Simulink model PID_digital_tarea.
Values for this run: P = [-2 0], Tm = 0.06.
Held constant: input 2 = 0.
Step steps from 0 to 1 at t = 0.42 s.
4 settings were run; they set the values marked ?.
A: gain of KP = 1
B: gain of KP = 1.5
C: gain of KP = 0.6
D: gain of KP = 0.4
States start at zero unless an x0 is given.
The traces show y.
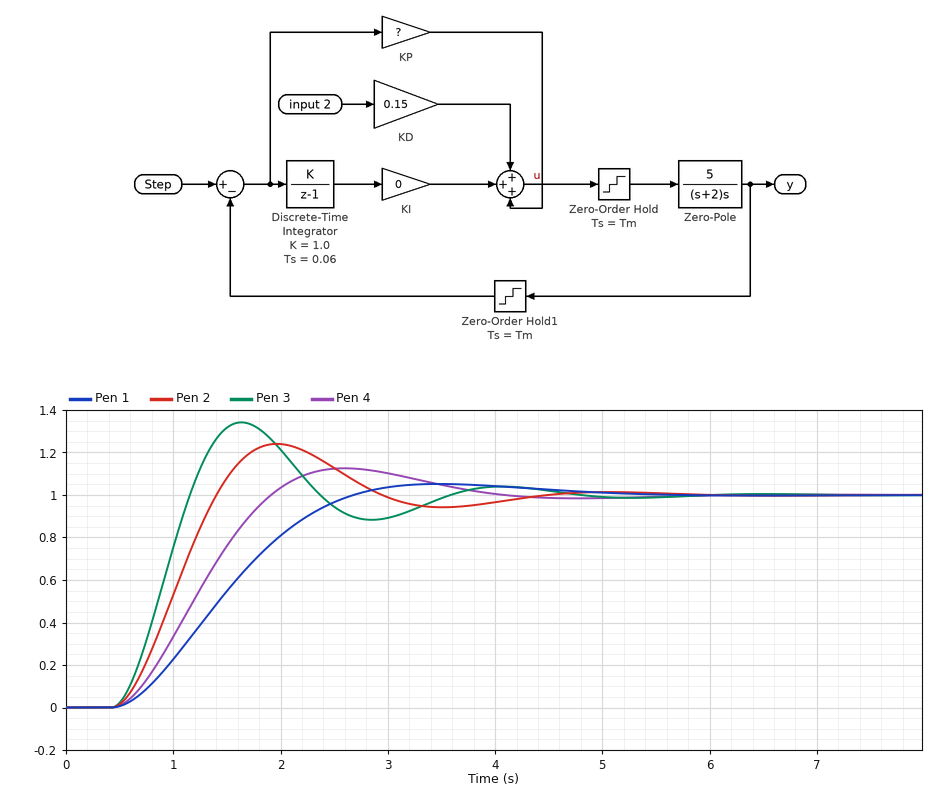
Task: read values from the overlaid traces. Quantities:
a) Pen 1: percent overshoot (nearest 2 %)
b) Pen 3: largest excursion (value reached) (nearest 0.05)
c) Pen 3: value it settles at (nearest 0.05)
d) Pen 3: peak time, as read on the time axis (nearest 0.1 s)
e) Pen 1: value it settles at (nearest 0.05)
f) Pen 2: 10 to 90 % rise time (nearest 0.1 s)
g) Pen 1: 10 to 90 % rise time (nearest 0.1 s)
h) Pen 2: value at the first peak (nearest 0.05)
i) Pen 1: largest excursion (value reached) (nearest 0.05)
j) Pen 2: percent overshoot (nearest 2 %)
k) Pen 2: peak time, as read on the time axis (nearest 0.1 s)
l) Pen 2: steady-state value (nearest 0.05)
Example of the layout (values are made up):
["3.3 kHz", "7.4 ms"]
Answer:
["6 %", "1.35", "1.00", "1.6 s", "1.00", "0.7 s", "1.5 s", "1.25", "1.05", "24 %", "2.0 s", "1.00"]
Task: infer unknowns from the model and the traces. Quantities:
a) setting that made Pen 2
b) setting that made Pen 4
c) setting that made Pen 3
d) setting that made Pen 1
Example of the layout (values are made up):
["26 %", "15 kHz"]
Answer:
["A", "C", "B", "D"]
